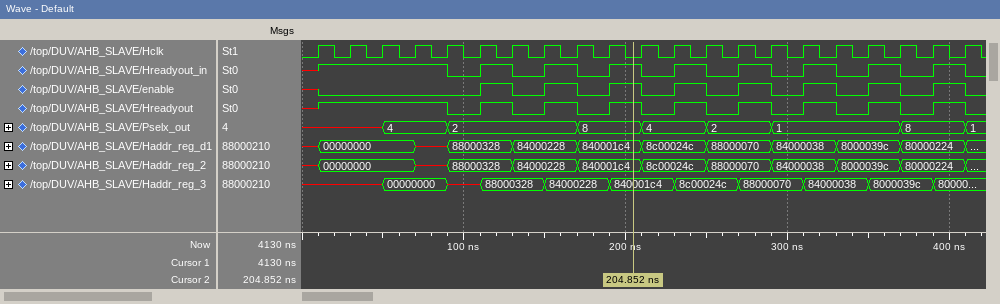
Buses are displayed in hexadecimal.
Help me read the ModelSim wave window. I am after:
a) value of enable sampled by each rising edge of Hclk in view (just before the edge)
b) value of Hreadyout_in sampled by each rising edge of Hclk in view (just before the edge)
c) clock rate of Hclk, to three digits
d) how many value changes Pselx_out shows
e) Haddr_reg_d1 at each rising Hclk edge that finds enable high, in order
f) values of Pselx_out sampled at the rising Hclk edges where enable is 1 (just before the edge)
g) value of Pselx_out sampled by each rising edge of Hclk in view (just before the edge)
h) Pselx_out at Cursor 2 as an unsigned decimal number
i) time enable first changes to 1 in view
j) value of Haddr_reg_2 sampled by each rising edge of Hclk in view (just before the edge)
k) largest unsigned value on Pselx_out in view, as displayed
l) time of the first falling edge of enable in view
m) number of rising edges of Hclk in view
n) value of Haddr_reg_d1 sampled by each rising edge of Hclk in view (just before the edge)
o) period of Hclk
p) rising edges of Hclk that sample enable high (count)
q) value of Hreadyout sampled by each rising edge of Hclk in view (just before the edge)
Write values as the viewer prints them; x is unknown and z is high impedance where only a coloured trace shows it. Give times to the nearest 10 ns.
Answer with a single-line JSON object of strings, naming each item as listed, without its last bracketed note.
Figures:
{"value of enable sampled by each rising edge of Hclk in view": "x 0 0 0 0 0 1 0 1 0 1 0 1 0 1 0 1 0 1 0 1", "value of Hreadyout_in sampled by each rising edge of Hclk in view": "x 1 1 1 1 0 1 0 1 0 1 0 1 0 1 0 1 0 1 0 1", "clock rate of Hclk, to three digits": "50.0 MHz", "how many value changes Pselx_out shows": "8", "Haddr_reg_d1 at each rising Hclk edge that finds enable high, in order": "88000328, 84000228, 840001c4, 8c00024c, 88000070, 84000038, 8000039c, 80000224", "values of Pselx_out sampled at the rising Hclk edges where enable is 1": "2, 2, 8, 4, 2, 1, 1, 8", "value of Pselx_out sampled by each rising edge of Hclk in view": "x, x, x, 4, 4, 2, 2, 2, 2, 8, 8, 4, 4, 2, 2, 1, 1, 1, 1, 8, 8", "Pselx_out at Cursor 2 as an unsigned decimal number": "8", "time enable first changes to 1 in view": "110 ns", "value of Haddr_reg_2 sampled by each rising edge of Hclk in view": "x, 00000000, 00000000, 00000000, x, 88000328, 88000328, 84000228, 84000228, 840001c4, 840001c4, 8c00024c, 8c00024c, 88000070, 88000070, 84000038, 84000038, 8000039c, 8000039c, 80000224, 80000224", "largest unsigned value on Pselx_out in view, as displayed": "8", "time of the first falling edge of enable in view": "130 ns", "number of rising edges of Hclk in view": "21", "value of Haddr_reg_d1 sampled by each rising edge of Hclk in view": "x, 00000000, 00000000, 00000000, x, 88000328, 88000328, 84000228, 84000228, 840001c4, 840001c4, 8c00024c, 8c00024c, 88000070, 88000070, 84000038, 84000038, 8000039c, 8000039c, 80000224, 80000224", "period of Hclk": "20 ns", "rising edges of Hclk that sample enable high": "8", "value of Hreadyout sampled by each rising edge of Hclk in view": "x 1 1 1 1 0 1 0 1 0 1 0 1 0 1 0 1 0 1 0 1"}
